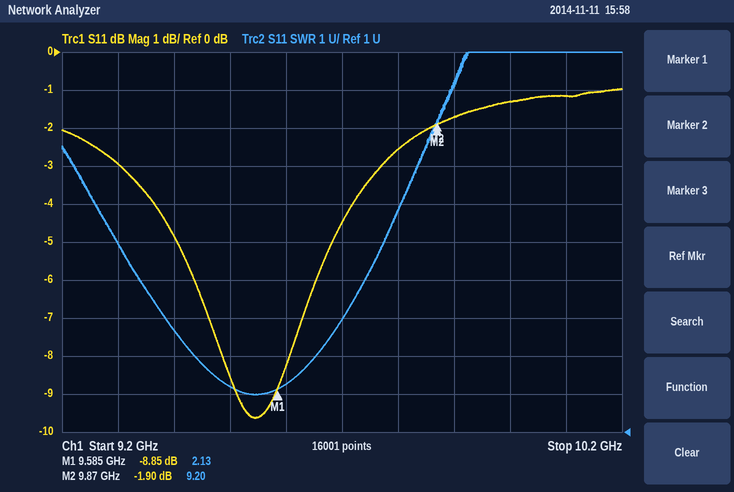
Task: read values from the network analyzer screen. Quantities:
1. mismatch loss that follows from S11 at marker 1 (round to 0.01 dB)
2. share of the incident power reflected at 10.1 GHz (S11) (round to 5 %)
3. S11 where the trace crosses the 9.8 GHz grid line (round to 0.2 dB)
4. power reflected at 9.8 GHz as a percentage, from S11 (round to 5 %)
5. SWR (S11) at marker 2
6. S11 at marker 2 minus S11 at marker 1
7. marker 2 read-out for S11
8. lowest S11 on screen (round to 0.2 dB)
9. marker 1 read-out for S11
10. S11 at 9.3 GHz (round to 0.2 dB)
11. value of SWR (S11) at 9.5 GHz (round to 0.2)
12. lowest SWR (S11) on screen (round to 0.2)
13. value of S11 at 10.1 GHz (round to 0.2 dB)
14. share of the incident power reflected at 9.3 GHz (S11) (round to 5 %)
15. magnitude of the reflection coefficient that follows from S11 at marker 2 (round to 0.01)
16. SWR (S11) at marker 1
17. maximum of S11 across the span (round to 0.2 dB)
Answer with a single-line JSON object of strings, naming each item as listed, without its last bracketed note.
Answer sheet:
{"mismatch loss that follows from S11 at marker 1": "0.61 dB", "share of the incident power reflected at 10.1 GHz (S11)": "75 %", "S11 where the trace crosses the 9.8 GHz grid line": "-2.6 dB", "power reflected at 9.8 GHz as a percentage, from S11": "55 %", "SWR (S11) at marker 2": "9.20", "S11 at marker 2 minus S11 at marker 1": "6.95 dB", "marker 2 read-out for S11": "-1.90 dB", "lowest S11 on screen": "-9.6 dB", "marker 1 read-out for S11": "-8.85 dB", "S11 at 9.3 GHz": "-3.0 dB", "value of SWR (S11) at 9.5 GHz": "2.2", "lowest SWR (S11) on screen": "2.0", "value of S11 at 10.1 GHz": "-1.2 dB", "share of the incident power reflected at 9.3 GHz (S11)": "50 %", "magnitude of the reflection coefficient that follows from S11 at marker 2": "0.80", "SWR (S11) at marker 1": "2.13", "maximum of S11 across the span": "-1.0 dB"}
